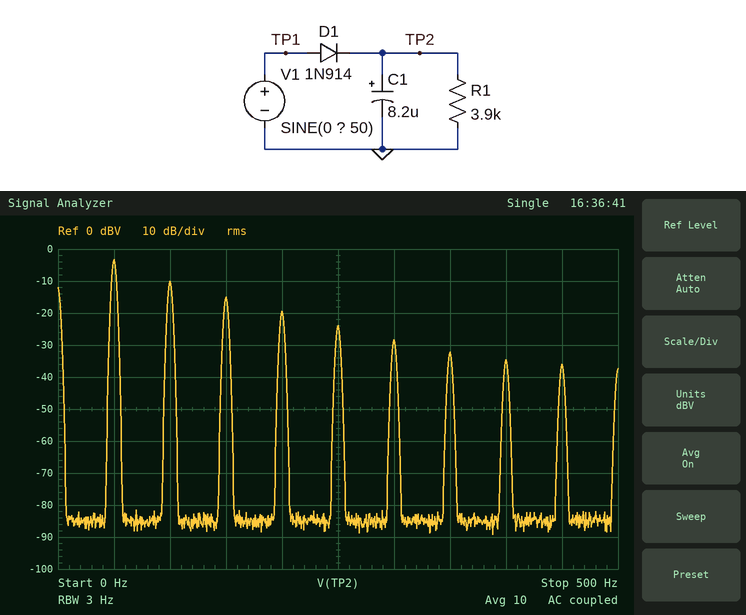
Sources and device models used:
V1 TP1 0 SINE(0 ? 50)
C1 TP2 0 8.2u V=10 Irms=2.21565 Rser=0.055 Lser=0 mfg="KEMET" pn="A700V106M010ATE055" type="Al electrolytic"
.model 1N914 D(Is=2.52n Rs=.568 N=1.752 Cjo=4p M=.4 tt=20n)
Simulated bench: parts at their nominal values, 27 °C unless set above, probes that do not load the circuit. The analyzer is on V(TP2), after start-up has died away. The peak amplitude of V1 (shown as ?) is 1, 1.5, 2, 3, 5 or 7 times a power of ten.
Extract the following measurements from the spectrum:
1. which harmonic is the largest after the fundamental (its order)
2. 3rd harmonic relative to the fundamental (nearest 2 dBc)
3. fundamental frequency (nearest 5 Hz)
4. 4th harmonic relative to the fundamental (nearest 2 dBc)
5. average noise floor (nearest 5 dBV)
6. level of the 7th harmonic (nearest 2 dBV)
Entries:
2
-12 dBc
50 Hz
-16 dBc
-85 dBV
-32 dBV
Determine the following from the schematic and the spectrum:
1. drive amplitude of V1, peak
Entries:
7 V
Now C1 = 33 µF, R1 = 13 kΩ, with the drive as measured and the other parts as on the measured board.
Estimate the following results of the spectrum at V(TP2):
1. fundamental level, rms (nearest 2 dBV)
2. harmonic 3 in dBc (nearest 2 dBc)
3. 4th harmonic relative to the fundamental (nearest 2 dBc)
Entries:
-24 dBV
-10 dBc
-12 dBc
